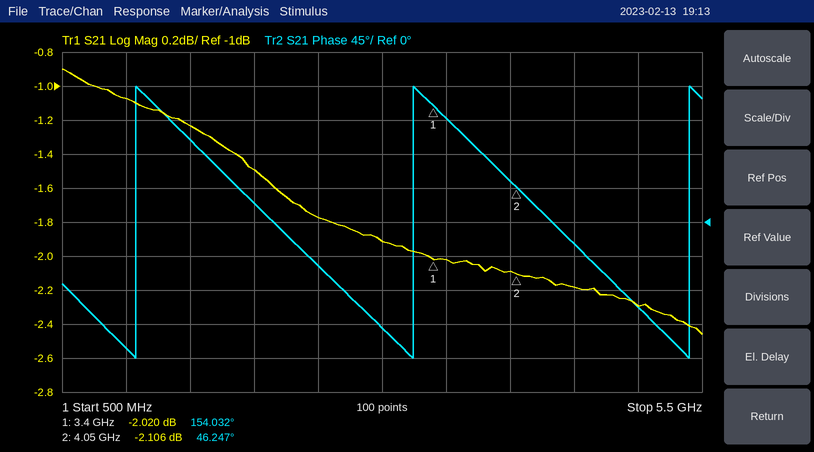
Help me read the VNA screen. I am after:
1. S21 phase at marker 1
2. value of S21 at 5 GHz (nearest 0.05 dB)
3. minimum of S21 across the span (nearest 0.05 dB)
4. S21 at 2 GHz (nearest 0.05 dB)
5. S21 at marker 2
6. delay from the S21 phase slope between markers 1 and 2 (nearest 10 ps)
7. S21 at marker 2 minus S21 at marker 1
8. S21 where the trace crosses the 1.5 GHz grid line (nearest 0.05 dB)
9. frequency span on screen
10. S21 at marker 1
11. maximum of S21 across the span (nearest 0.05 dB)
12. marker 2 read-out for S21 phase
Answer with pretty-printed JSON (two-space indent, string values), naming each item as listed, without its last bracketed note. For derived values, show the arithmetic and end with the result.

{
  "S21 phase at marker 1": "154.032°",
  "value of S21 at 5 GHz": "-2.30 dB",
  "minimum of S21 across the span": "-2.45 dB",
  "S21 at 2 GHz": "-1.50 dB",
  "S21 at marker 2": "-2.106 dB",
  "delay from the S21 phase slope between markers 1 and 2": "−(46.247° − (154.032°))/(360° × 650 MHz) ≈ 461 ps, so 460 ps to the nearest 10 ps",
  "S21 at marker 2 minus S21 at marker 1": "-2.106 − (-2.02) = -0.086 dB",
  "S21 where the trace crosses the 1.5 GHz grid line": "-1.25 dB",
  "frequency span on screen": "5 GHz",
  "S21 at marker 1": "-2.020 dB",
  "maximum of S21 across the span": "-0.90 dB",
  "marker 2 read-out for S21 phase": "46.247°"
}
